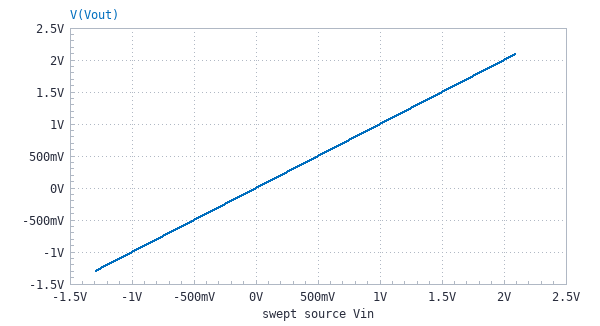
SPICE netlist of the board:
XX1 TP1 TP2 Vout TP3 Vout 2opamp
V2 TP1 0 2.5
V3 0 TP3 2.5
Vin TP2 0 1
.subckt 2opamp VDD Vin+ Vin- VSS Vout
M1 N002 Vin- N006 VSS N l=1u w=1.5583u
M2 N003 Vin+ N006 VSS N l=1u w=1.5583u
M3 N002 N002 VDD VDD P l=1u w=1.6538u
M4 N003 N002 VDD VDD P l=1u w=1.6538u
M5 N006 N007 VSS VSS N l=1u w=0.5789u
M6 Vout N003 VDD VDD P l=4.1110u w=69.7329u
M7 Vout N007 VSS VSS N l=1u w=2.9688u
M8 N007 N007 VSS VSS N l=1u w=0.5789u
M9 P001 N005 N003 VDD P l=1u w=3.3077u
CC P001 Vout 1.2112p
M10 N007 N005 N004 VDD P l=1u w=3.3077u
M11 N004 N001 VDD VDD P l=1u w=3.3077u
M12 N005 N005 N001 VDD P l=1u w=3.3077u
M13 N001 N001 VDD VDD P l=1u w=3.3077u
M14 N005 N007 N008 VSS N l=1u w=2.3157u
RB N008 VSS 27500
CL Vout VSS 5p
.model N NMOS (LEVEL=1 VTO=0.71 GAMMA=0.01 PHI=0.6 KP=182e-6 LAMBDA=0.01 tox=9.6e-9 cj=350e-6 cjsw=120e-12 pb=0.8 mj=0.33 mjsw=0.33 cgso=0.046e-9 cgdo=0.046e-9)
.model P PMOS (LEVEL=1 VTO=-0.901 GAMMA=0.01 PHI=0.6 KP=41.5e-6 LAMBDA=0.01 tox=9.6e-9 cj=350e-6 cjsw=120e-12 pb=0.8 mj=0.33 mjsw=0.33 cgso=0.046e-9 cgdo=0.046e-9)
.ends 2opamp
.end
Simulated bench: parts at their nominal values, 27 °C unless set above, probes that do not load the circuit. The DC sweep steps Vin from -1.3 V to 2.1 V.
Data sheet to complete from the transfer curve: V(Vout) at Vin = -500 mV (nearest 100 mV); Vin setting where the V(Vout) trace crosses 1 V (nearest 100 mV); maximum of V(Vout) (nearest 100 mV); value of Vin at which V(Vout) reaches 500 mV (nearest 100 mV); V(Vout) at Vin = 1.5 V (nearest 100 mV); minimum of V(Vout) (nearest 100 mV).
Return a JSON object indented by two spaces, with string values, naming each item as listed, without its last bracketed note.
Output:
{
  "V(Vout) at Vin = -500 mV": "-500 mV",
  "Vin setting where the V(Vout) trace crosses 1 V": "1.0 V",
  "maximum of V(Vout)": "2.1 V",
  "value of Vin at which V(Vout) reaches 500 mV": "500 mV",
  "V(Vout) at Vin = 1.5 V": "1.5 V",
  "minimum of V(Vout)": "-1.3 V"
}
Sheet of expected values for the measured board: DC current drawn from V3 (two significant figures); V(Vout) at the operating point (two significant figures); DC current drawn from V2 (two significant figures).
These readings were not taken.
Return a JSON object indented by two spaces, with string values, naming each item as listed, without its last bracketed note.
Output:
{
  "DC current drawn from V3": "51 µA",
  "V(Vout) at the operating point": "1.0 V",
  "DC current drawn from V2": "51 µA"
}
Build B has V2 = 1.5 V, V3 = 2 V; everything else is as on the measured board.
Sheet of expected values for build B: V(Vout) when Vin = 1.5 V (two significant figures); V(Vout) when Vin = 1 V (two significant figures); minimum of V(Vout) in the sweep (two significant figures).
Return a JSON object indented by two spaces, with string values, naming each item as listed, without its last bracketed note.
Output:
{
  "V(Vout) when Vin = 1.5 V": "1.3 V",
  "V(Vout) when Vin = 1 V": "1.0 V",
  "minimum of V(Vout) in the sweep": "-2.0 V"
}
